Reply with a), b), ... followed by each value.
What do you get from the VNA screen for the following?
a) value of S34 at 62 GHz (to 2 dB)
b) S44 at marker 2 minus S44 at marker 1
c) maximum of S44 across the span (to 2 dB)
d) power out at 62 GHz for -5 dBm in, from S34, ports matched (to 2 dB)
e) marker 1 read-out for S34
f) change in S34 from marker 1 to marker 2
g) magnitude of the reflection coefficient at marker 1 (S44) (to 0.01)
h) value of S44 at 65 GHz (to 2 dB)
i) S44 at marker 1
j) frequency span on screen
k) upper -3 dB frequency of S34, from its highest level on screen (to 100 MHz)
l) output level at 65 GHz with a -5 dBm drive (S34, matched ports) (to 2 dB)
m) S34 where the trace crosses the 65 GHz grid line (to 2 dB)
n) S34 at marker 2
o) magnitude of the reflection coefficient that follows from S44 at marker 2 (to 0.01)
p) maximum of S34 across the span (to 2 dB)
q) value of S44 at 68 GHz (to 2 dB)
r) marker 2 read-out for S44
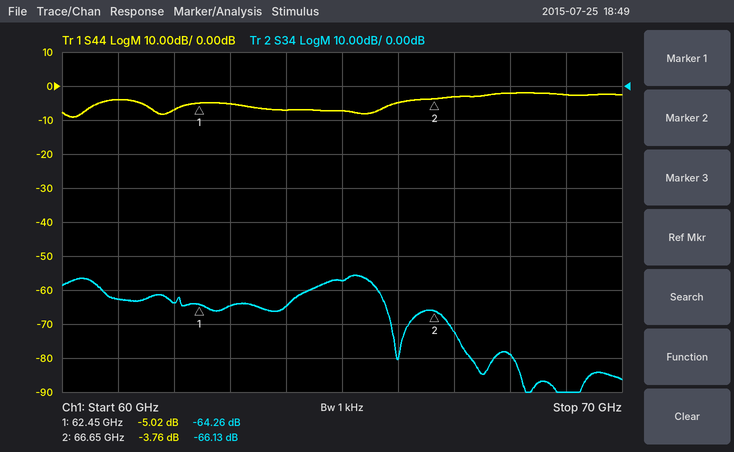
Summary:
a) -64 dB
b) 1.26 dB
c) -2 dB
d) -68 dBm
e) -64.26 dB
f) -1.87 dB
g) 0.56
h) -8 dB
i) -5.02 dB
j) 10 GHz
k) 65.6 GHz
l) -62 dBm
m) -58 dB
n) -66.13 dB
o) 0.65
p) -56 dB
q) -2 dB
r) -3.76 dB
